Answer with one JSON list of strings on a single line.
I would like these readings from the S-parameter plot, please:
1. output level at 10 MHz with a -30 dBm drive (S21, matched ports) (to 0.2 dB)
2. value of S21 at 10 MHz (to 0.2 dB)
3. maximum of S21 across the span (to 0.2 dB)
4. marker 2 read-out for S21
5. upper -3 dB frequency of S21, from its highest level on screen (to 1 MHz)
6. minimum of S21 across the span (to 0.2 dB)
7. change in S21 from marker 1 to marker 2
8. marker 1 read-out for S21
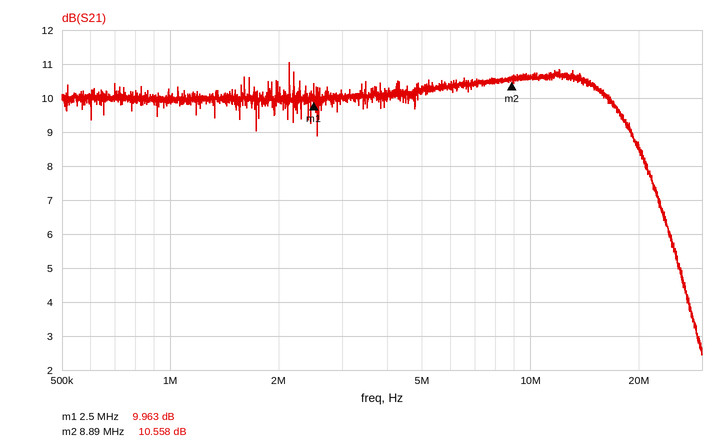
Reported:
["-19.4 dBm", "10.6 dB", "11.0 dB", "10.558 dB", "21 MHz", "2.4 dB", "0.595 dB", "9.963 dB"]
